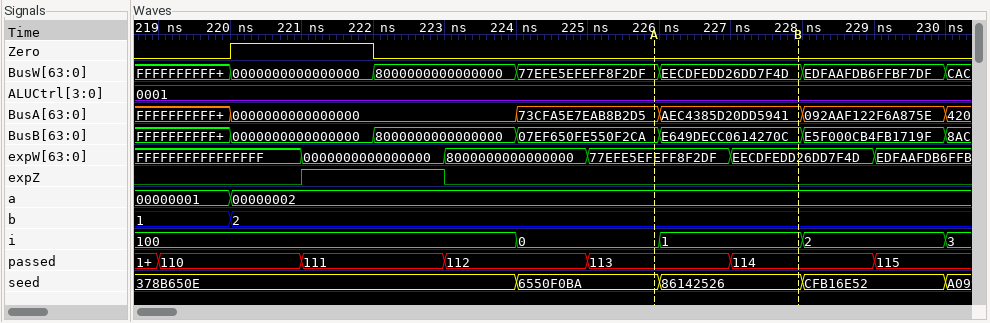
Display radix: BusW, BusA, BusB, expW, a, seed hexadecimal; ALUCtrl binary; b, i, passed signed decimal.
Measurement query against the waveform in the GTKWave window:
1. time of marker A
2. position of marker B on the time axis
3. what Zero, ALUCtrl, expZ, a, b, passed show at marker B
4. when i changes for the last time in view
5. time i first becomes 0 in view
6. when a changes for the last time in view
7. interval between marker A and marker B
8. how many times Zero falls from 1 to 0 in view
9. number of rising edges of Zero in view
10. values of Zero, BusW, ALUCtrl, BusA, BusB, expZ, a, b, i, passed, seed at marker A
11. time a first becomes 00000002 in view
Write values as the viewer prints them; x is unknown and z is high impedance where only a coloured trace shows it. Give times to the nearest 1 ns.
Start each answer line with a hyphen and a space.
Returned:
- 226 ns
- 228 ns
- Zero=0, ALUCtrl=0001, expZ=0, a=00000002, b=2, passed=114
- 230 ns
- 224 ns
- 220 ns
- 2 ns
- 1
- 1
- Zero=0, BusW=77EFE5EFEFF8F2DF, ALUCtrl=0001, BusA=73CFA5E7EAB8B2D5, BusB=07EF650FE550F2CA, expZ=0, a=00000002, b=2, i=0, passed=113, seed=6550F0BA
- 220 ns
